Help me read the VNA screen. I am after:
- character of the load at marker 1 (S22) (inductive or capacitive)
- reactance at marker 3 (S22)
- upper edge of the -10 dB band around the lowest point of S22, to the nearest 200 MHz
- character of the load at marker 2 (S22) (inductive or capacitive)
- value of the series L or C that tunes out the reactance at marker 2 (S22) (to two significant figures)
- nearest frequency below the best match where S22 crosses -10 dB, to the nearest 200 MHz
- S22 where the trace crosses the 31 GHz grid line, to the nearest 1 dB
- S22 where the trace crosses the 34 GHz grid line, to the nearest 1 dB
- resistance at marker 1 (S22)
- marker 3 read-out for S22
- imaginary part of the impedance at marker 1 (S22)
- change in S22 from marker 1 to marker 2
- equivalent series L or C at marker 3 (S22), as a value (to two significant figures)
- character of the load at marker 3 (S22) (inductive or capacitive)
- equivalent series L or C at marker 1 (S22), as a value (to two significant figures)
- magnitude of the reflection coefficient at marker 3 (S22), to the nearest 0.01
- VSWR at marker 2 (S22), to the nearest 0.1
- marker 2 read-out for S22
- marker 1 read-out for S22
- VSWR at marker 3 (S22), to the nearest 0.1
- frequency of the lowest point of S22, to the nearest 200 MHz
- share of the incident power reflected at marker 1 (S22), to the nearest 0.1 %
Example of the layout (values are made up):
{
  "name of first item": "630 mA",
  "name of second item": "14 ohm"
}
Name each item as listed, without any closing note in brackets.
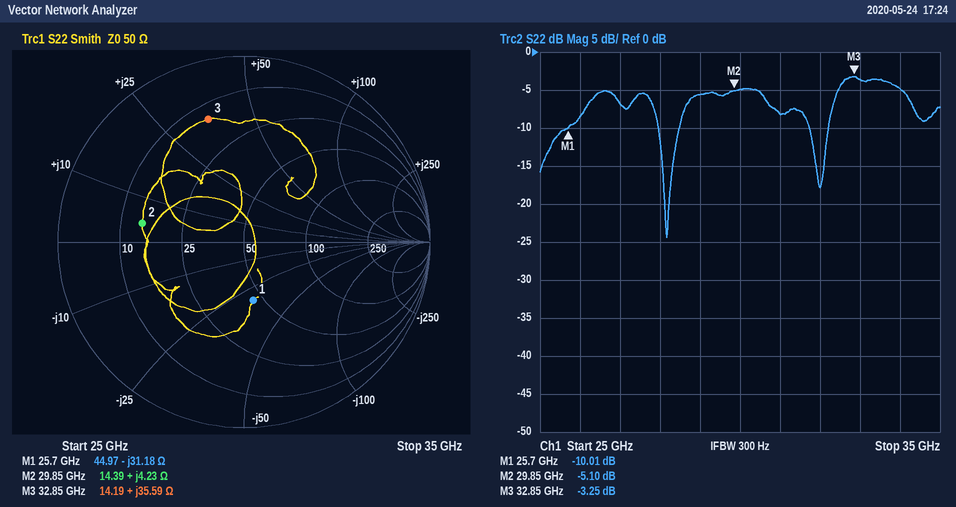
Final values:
{
  "character of the load at marker 1 (S22)": "capacitive",
  "reactance at marker 3": "+35.59 Ω",
  "upper edge of the -10 dB band around the lowest point of S22, to the nearest 200 MHz": "28.4 GHz",
  "character of the load at marker 2 (S22)": "inductive",
  "value of the series L or C that tunes out the reactance at marker 2 (S22)": "1.3 pF",
  "nearest frequency below the best match where S22 crosses -10 dB, to the nearest 200 MHz": "28.0 GHz",
  "S22 where the trace crosses the 31 GHz grid line, to the nearest 1 dB": "-8 dB",
  "S22 where the trace crosses the 34 GHz grid line, to the nearest 1 dB": "-5 dB",
  "resistance at marker 1": "44.97 Ω",
  "marker 3 read-out for S22": "-3.25 dB",
  "imaginary part of the impedance at marker 1": "-31.18 Ω",
  "change in S22 from marker 1 to marker 2": "4.91 dB",
  "equivalent series L or C at marker 3 (S22), as a value": "170 pH",
  "character of the load at marker 3 (S22)": "inductive",
  "equivalent series L or C at marker 1 (S22), as a value": "200 fF",
  "magnitude of the reflection coefficient at marker 3 (S22), to the nearest 0.01": "0.69",
  "VSWR at marker 2 (S22), to the nearest 0.1": "3.5",
  "marker 2 read-out for S22": "-5.10 dB",
  "marker 1 read-out for S22": "-10.01 dB",
  "VSWR at marker 3 (S22), to the nearest 0.1": "5.4",
  "frequency of the lowest point of S22, to the nearest 200 MHz": "28.2 GHz",
  "share of the incident power reflected at marker 1 (S22), to the nearest 0.1 %": "10.0 %"
}
